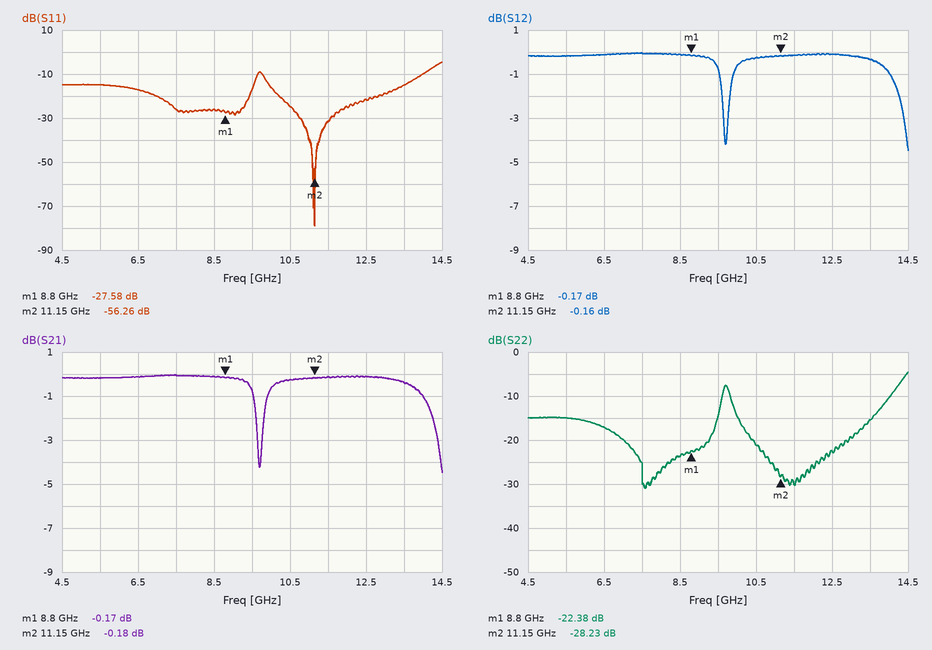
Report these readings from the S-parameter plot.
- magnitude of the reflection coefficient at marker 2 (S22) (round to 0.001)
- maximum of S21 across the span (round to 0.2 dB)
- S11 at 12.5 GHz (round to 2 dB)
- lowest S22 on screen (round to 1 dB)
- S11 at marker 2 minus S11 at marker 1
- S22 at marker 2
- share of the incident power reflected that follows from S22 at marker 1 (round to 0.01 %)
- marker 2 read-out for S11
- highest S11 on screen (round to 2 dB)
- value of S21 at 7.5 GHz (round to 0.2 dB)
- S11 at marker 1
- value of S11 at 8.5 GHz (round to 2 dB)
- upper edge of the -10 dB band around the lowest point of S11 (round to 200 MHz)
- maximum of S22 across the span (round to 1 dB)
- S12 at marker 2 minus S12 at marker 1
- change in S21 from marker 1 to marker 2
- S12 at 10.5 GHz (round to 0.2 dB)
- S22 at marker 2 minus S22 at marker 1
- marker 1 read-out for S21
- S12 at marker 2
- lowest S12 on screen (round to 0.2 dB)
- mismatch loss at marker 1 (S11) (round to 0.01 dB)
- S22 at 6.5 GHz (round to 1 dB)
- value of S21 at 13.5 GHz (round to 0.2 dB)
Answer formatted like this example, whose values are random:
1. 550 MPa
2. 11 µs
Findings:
1. 0.039
2. 0.0 dB
3. -22 dB
4. -31 dB
5. -28.68 dB
6. -28.23 dB
7. 0.58 %
8. -56.26 dB
9. -4 dB
10. 0.0 dB
11. -27.58 dB
12. -26 dB
13. 14.0 GHz
14. -5 dB
15. 0.01 dB
16. -0.01 dB
17. -0.2 dB
18. -5.85 dB
19. -0.17 dB
20. -0.16 dB
21. -4.4 dB
22. 0.01 dB
23. -17 dB
24. -0.4 dB
